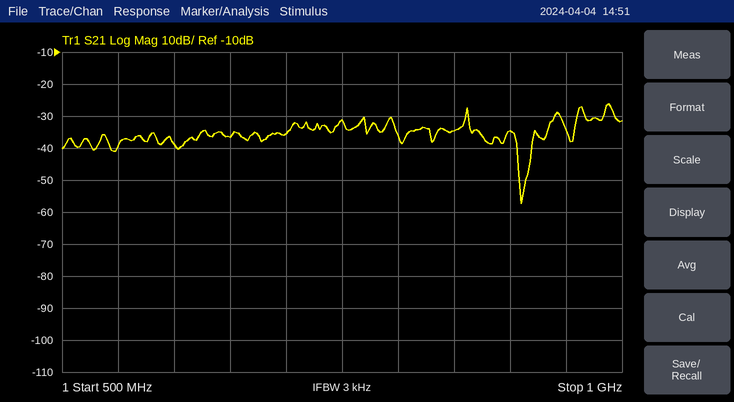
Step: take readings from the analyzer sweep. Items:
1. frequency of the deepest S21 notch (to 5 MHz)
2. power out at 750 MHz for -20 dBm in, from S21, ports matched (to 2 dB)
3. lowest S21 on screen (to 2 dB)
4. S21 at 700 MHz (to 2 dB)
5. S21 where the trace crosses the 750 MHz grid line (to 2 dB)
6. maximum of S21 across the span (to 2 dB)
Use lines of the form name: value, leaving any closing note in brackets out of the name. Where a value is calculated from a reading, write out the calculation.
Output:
frequency of the deepest S21 notch: 910 MHz
power out at 750 MHz for -20 dBm in, from S21, ports matched: -20 dBm + (-32 dB) = -52 dBm
lowest S21 on screen: -58 dB
S21 at 700 MHz: -36 dB
S21 where the trace crosses the 750 MHz grid line: -32 dB
maximum of S21 across the span: -26 dB
